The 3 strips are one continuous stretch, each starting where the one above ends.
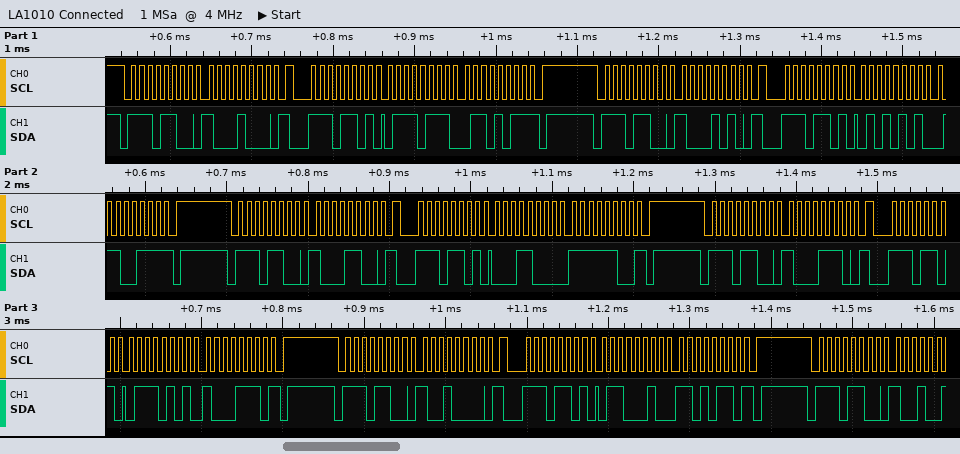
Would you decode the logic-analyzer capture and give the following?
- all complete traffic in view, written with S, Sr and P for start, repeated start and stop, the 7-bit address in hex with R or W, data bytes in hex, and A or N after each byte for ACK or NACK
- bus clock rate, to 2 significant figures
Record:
S 76W A 88 A Sr 76R A 77 A 6B N P S 76W A 8A A Sr 76R A 55 A 67 N P S 76W A 8C A Sr 76R A 18 A FC N P S 76W A 8E A Sr 76R A 75 A 8E N P S 76W A 90 A Sr 76R A 62 A D6 N P S 76W A
100 kHz
